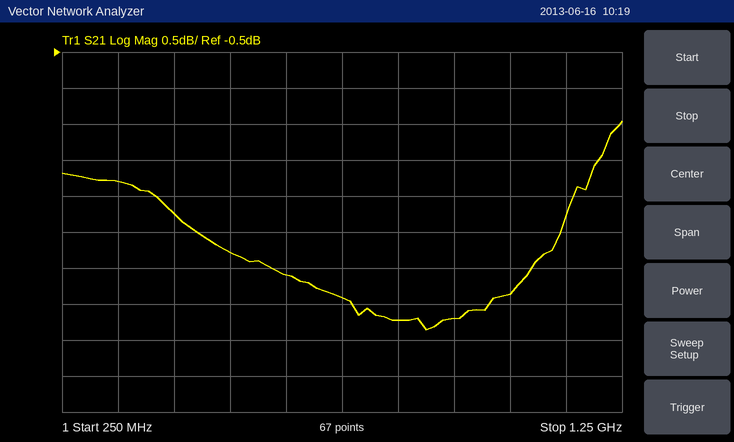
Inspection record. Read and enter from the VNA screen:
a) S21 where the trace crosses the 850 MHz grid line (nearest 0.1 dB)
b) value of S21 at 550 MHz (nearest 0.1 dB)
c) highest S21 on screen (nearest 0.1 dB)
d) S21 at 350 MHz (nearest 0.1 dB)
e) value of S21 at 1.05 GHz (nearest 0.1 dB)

-4.2 dB
-3.3 dB
-1.5 dB
-2.3 dB
-3.9 dB
